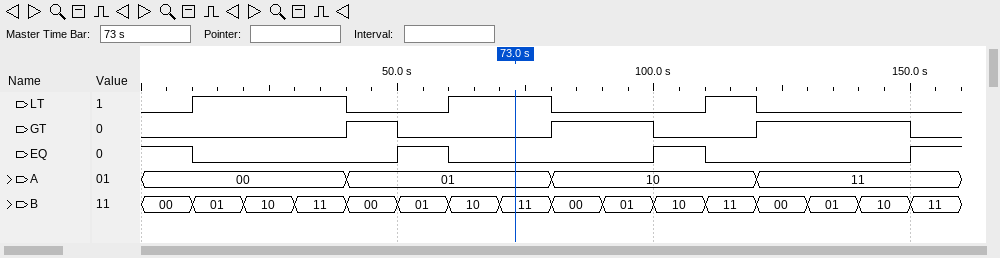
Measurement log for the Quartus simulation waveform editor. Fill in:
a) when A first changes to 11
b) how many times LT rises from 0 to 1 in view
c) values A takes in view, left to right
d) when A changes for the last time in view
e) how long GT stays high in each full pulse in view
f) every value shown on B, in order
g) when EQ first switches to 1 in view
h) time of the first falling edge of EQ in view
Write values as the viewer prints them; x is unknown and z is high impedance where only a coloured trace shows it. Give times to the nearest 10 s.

120 s
3
00, 01, 10, 11
120 s
10 s, 20 s, 30 s
00, 01, 10, 11, 00, 01, 10, 11, 00, 01, 10, 11, 00, 01, 10, 11
50 s
10 s
